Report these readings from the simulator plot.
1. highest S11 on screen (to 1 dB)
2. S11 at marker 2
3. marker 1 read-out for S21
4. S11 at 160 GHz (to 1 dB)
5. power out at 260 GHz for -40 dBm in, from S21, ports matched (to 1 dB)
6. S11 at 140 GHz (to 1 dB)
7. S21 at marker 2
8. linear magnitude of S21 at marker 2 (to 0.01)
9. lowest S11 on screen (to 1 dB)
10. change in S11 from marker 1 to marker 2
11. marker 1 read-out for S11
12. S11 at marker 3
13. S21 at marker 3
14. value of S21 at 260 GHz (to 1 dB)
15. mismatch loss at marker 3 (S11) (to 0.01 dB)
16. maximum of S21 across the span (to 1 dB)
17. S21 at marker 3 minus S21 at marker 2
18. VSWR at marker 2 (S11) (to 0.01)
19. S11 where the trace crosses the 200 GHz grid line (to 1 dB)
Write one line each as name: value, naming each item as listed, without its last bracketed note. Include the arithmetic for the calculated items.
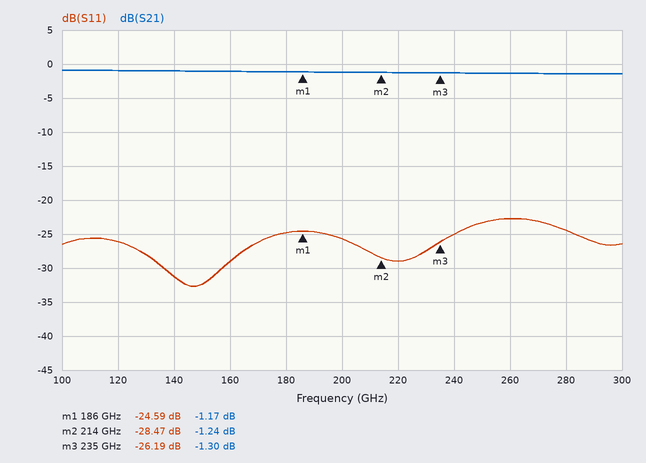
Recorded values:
highest S11 on screen: -23 dB
S11 at marker 2: -28.47 dB
marker 1 read-out for S21: -1.17 dB
S11 at 160 GHz: -29 dB
power out at 260 GHz for -40 dBm in, from S21, ports matched: -40 dBm + (-1 dB) = -41 dBm
S11 at 140 GHz: -31 dB
S21 at marker 2: -1.24 dB
linear magnitude of S21 at marker 2: 10^(-1.24/20) ≈ 0.87
lowest S11 on screen: -33 dB
change in S11 from marker 1 to marker 2: -28.47 − (-24.59) = -3.88 dB
marker 1 read-out for S11: -24.59 dB
S11 at marker 3: -26.19 dB
S21 at marker 3: -1.30 dB
value of S21 at 260 GHz: -1 dB
mismatch loss at marker 3 (S11): −10 log10(1 − 10^(-26.19/10)) ≈ 0.01 dB
maximum of S21 across the span: -1 dB
S21 at marker 3 minus S21 at marker 2: -1.3 − (-1.24) = -0.06 dB
VSWR at marker 2 (S11): (1 + 0.0377)/(1 − 0.0377) ≈ 1.08
S11 where the trace crosses the 200 GHz grid line: -26 dB
